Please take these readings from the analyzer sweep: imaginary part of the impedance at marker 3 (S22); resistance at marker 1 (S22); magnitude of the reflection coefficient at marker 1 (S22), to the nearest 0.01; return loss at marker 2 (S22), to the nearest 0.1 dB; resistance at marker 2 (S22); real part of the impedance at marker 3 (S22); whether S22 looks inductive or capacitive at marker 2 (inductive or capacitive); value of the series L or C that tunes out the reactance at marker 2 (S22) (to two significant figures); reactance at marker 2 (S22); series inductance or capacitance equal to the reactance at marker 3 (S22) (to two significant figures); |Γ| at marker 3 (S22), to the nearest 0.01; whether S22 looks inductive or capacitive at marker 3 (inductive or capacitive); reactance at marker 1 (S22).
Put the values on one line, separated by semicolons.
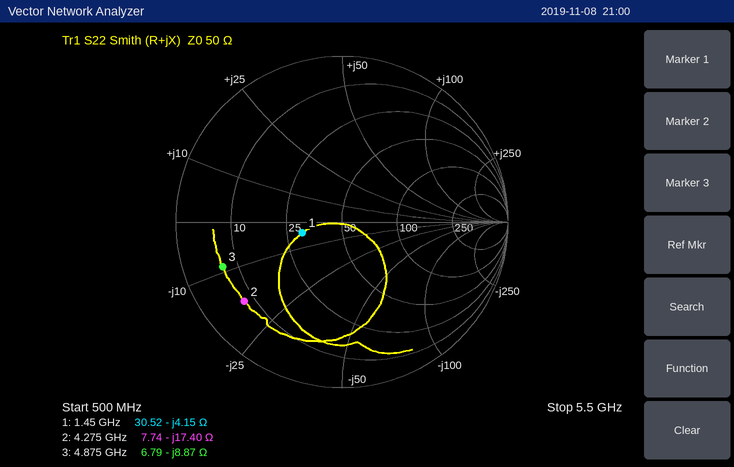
-8.87 Ω; 30.52 Ω; 0.25; 2.4 dB; 7.74 Ω; 6.79 Ω; capacitive; 650 pH; -17.40 Ω; 3.7 pF; 0.77; capacitive; -4.15 Ω
